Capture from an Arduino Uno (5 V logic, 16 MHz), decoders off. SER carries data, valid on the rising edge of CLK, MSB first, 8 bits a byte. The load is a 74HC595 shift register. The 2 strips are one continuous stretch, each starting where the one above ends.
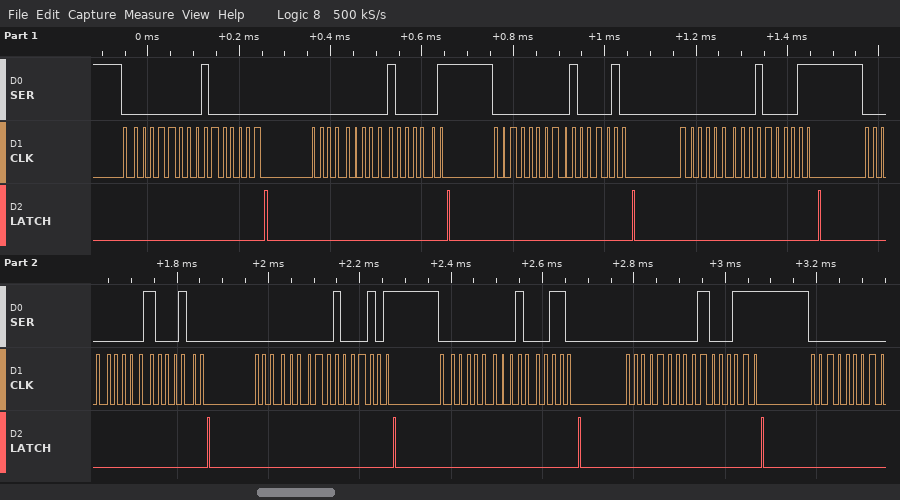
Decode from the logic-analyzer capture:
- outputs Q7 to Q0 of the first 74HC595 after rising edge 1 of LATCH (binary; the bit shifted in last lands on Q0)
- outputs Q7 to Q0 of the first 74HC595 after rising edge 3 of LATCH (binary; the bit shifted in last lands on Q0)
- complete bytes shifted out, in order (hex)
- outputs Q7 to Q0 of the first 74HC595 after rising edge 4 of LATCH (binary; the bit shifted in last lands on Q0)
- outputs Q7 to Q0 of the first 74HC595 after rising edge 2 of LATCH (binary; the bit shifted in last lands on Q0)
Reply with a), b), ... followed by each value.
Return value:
a) 01000000
b) 01000010
c) 00 40 00 41 00 42 00 43 00 44 00 45 00 46 00 47 00
d) 01000011
e) 01000001
